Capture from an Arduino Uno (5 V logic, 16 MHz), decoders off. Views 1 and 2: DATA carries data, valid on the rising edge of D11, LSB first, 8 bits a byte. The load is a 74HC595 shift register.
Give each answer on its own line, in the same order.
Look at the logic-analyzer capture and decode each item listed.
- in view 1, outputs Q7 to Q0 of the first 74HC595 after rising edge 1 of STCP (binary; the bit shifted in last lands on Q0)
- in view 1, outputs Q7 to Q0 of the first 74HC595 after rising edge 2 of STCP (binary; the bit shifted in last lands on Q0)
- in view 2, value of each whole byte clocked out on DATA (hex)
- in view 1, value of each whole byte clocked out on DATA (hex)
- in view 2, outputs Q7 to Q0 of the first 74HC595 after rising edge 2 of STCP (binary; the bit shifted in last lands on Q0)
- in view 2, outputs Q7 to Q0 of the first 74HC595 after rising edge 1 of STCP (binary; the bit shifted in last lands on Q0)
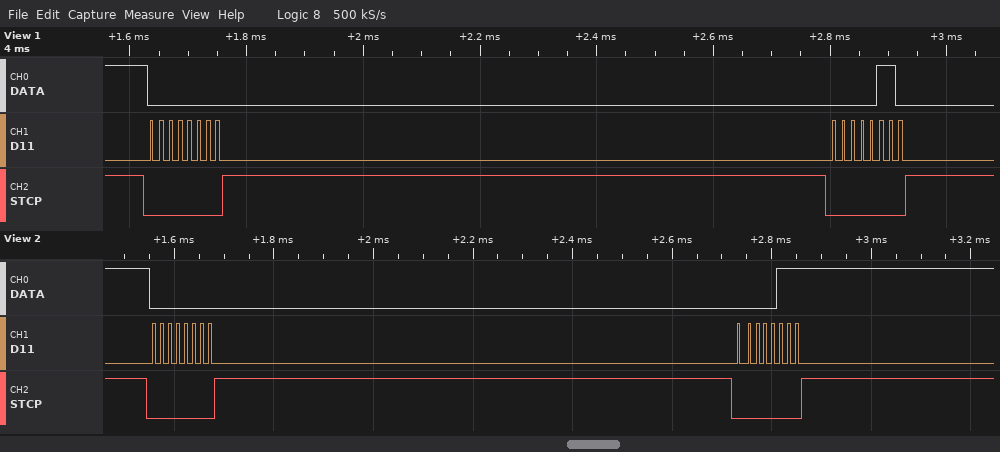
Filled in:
00000000
00000110
00 E0
00 60
00000111
00000000
